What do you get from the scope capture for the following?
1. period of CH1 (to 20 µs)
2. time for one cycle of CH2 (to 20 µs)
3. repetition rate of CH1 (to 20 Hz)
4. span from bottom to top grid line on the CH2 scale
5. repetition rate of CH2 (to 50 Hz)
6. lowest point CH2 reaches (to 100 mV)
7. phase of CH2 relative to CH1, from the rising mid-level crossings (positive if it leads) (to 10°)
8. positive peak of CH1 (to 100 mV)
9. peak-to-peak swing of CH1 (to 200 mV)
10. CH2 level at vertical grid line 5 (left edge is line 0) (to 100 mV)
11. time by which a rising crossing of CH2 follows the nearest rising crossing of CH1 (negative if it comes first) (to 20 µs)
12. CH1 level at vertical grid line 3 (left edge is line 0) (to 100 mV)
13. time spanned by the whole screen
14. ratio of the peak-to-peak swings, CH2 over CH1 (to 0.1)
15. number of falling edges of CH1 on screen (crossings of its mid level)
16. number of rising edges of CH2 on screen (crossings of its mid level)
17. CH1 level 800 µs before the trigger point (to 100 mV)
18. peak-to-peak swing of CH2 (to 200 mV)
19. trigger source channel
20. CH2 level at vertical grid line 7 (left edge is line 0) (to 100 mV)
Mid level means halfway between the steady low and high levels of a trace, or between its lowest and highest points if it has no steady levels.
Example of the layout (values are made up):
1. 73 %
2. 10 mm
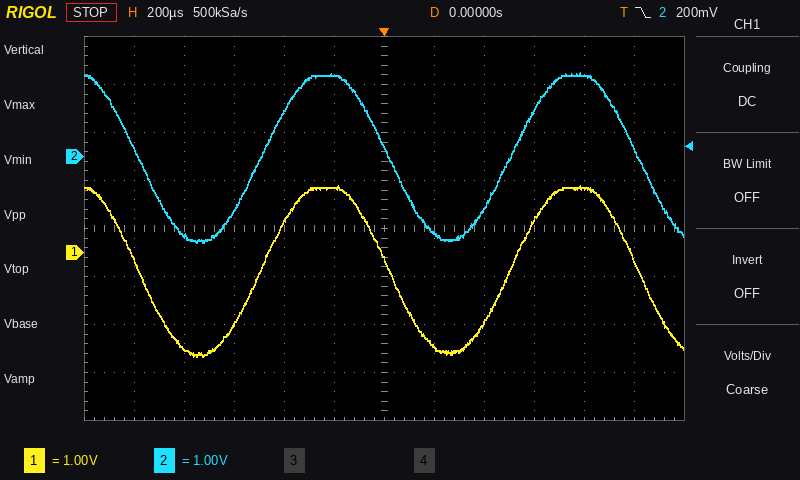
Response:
1. 1.00 ms
2. 1.00 ms
3. 1.00 kHz
4. 8 V
5. 1.00 kHz
6. -1.8 V
7. 0°
8. 1.4 V
9. 3.6 V
10. 1.7 V
11. 0 µs
12. -1.5 V
13. 2.4 ms
14. 1.0
15. 3
16. 2
17. -2.0 V
18. 3.6 V
19. CH2
20. -1.6 V
